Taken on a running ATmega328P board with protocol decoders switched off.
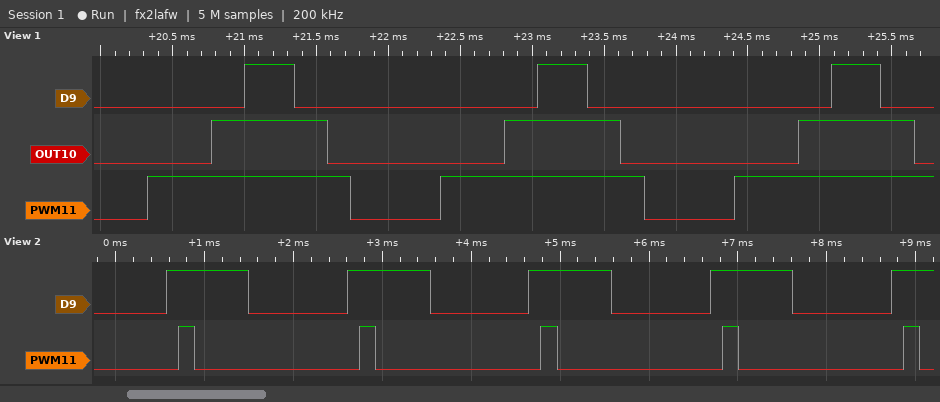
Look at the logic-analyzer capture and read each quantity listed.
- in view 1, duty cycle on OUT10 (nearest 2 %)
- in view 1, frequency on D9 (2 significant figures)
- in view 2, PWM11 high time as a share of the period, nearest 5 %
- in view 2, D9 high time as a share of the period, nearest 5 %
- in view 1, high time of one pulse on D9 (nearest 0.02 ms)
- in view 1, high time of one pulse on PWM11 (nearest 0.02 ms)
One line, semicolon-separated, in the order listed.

40 %; 490 Hz; 10 %; 45 %; 0.34 ms; 1.42 ms
